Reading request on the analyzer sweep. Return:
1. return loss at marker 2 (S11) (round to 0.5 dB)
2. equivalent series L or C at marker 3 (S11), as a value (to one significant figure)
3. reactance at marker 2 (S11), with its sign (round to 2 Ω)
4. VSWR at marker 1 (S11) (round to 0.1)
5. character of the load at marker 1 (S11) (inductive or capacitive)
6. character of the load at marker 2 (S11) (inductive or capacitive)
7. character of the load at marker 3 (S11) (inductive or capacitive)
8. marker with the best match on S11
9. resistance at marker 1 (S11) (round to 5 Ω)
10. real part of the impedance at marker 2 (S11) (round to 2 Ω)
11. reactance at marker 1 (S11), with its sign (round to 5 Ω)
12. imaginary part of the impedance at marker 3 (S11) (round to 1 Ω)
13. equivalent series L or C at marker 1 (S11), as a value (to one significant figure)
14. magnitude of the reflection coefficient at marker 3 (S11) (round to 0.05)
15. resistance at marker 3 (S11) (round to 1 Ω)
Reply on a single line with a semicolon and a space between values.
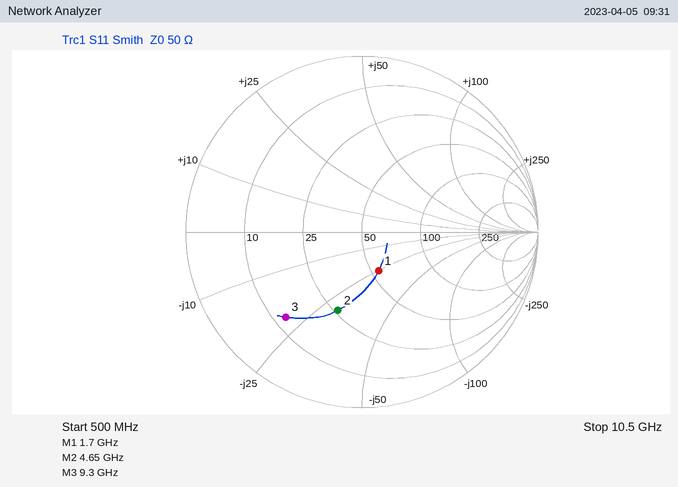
6.5 dB; 800 fF; -30 Ω; 1.6; capacitive; capacitive; capacitive; marker 1; 55 Ω; 26 Ω; -25 Ω; -21 Ω; 4 pF; 0.65; 13 Ω
